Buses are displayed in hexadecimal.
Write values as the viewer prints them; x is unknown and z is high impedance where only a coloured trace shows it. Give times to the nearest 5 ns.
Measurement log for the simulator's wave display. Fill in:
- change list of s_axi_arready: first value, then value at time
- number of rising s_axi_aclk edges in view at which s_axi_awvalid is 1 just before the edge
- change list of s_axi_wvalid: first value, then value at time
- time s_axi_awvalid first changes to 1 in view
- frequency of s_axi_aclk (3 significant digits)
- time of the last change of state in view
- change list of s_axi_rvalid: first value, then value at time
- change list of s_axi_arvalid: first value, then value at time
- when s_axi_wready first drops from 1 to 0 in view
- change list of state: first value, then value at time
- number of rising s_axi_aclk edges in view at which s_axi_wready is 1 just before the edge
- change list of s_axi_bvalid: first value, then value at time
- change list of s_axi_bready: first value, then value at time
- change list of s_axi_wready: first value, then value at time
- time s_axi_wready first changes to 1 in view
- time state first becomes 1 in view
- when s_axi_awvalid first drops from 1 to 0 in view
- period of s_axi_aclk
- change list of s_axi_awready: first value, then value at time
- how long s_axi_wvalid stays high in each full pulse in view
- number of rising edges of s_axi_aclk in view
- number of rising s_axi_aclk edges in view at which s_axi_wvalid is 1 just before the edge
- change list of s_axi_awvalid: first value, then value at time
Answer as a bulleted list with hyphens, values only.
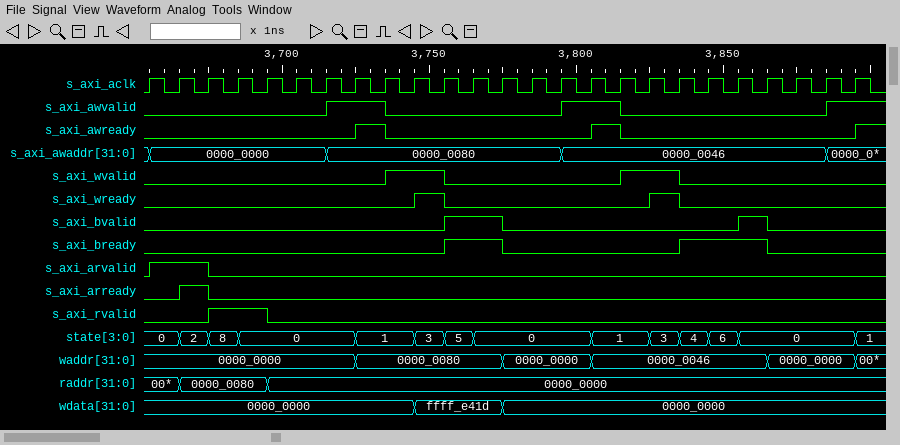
- 0, 1 at 3665 ns, 0 at 3675 ns
- 5
- 0, 1 at 3735 ns, 0 at 3755 ns, 1 at 3815 ns, 0 at 3835 ns
- 3715 ns
- 100 MHz
- 3895 ns
- 0, 1 at 3675 ns, 0 at 3695 ns
- 0, 1 at 3655 ns, 0 at 3675 ns
- 3755 ns
- 0, 2 at 3665 ns, 8 at 3675 ns, 0 at 3685 ns, 1 at 3725 ns, 3 at 3745 ns, 5 at 3755 ns, 0 at 3765 ns, 1 at 3805 ns, 3 at 3825 ns, 4 at 3835 ns, 6 at 3845 ns, 0 at 3855 ns, 1 at 3895 ns
- 2
- 0, 1 at 3755 ns, 0 at 3775 ns, 1 at 3855 ns, 0 at 3865 ns
- 0, 1 at 3755 ns, 0 at 3775 ns, 1 at 3835 ns, 0 at 3865 ns
- 0, 1 at 3745 ns, 0 at 3755 ns, 1 at 3825 ns, 0 at 3835 ns
- 3745 ns
- 3725 ns
- 3735 ns
- 10 ns
- 0, 1 at 3725 ns, 0 at 3735 ns, 1 at 3805 ns, 0 at 3815 ns, 1 at 3895 ns
- 20 ns, 20 ns
- 25
- 4
- 0, 1 at 3715 ns, 0 at 3735 ns, 1 at 3795 ns, 0 at 3815 ns, 1 at 3885 ns
